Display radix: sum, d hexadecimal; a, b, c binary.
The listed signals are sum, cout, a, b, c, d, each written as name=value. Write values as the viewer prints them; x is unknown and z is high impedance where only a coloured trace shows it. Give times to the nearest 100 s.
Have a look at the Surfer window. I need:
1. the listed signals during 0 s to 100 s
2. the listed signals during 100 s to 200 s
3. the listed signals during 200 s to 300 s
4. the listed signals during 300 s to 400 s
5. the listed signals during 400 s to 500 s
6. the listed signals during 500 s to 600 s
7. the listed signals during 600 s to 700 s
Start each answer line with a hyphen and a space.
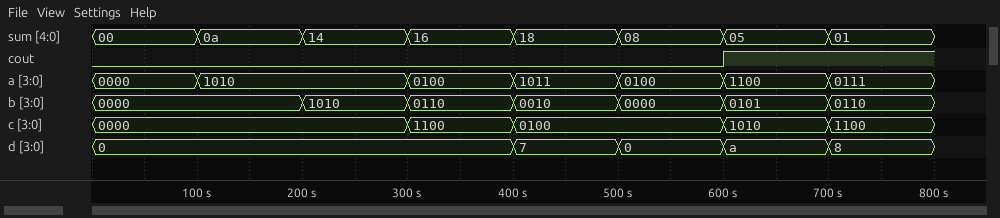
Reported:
- sum=00, cout=0, a=0000, b=0000, c=0000, d=0
- sum=0a, cout=0, a=1010, b=0000, c=0000, d=0
- sum=14, cout=0, a=1010, b=1010, c=0000, d=0
- sum=16, cout=0, a=0100, b=0110, c=1100, d=0
- sum=18, cout=0, a=1011, b=0010, c=0100, d=7
- sum=08, cout=0, a=0100, b=0000, c=0100, d=0
- sum=05, cout=1, a=1100, b=0101, c=1010, d=a
